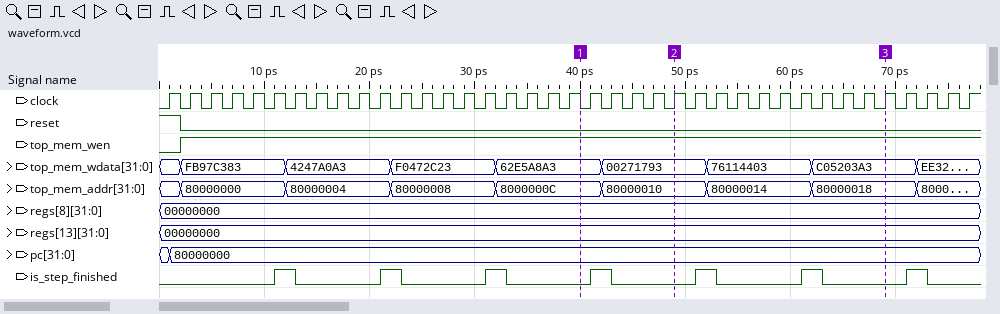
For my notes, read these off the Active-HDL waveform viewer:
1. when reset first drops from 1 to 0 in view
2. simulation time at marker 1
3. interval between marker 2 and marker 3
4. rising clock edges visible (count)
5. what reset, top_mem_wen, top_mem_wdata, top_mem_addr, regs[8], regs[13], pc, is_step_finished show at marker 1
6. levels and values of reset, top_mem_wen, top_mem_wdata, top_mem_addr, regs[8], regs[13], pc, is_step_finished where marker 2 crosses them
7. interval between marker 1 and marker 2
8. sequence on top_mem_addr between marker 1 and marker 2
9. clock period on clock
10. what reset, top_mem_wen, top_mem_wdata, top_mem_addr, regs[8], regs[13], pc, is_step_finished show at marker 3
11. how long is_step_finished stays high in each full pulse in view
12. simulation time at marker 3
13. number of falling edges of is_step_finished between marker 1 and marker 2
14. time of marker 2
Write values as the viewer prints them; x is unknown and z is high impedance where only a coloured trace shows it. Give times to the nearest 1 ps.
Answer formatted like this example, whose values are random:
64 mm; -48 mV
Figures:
2 ps; 40 ps; 20 ps; 39; reset=0, top_mem_wen=1, top_mem_wdata=62E5A8A3, top_mem_addr=8000000C, regs[8]=00000000, regs[13]=00000000, pc=80000000, is_step_finished=0; reset=0, top_mem_wen=1, top_mem_wdata=00271793, top_mem_addr=80000010, regs[8]=00000000, regs[13]=00000000, pc=80000000, is_step_finished=0; 9 ps; 8000000C, 80000010; 2 ps; reset=0, top_mem_wen=1, top_mem_wdata=C05203A3, top_mem_addr=80000018, regs[8]=00000000, regs[13]=00000000, pc=80000000, is_step_finished=0; 2 ps, 2 ps, 2 ps, 2 ps, 2 ps, 2 ps, 2 ps; 69 ps; 1; 49 ps
